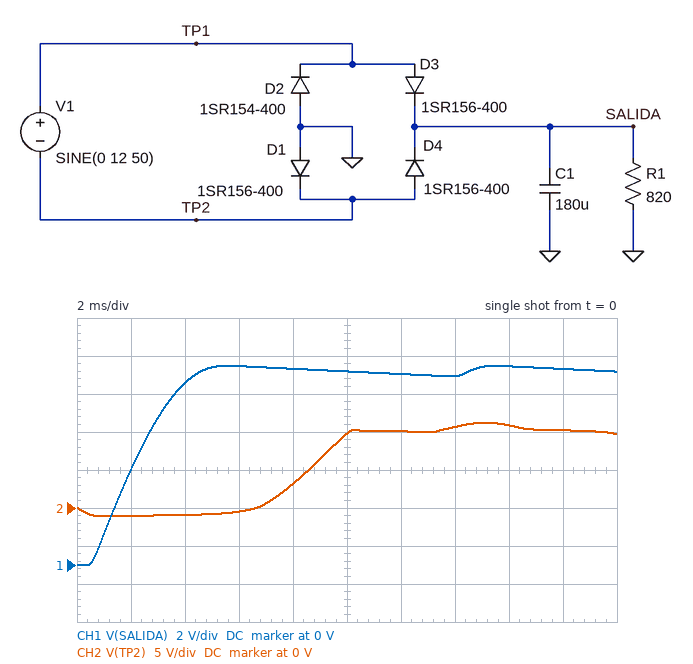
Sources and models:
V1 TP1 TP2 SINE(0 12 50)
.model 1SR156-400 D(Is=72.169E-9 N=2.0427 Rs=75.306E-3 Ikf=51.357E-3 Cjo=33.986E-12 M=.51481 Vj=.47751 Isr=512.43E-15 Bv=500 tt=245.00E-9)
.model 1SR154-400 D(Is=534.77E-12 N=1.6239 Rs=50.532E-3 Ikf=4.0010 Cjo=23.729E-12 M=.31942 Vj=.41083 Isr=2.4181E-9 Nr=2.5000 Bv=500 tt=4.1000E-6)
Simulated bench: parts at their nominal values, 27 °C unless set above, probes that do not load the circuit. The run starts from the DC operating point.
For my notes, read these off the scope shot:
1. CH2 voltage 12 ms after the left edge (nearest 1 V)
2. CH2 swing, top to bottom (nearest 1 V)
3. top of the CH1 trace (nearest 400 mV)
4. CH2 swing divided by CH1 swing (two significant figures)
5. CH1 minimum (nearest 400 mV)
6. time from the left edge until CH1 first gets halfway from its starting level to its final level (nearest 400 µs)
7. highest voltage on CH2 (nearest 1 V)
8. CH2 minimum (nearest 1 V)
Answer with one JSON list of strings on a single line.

["10 V", "12 V", "10.4 V", "1.2", "0 V", "2.0 ms", "11 V", "-1 V"]
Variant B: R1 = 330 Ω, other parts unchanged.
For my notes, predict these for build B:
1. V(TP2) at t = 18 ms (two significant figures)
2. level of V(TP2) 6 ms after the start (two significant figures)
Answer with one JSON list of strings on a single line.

["9.9 V", "-520 mV"]
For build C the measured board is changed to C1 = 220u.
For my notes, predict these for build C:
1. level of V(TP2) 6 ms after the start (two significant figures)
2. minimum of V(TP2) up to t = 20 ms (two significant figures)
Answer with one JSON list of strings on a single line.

["-480 mV", "-1.1 V"]
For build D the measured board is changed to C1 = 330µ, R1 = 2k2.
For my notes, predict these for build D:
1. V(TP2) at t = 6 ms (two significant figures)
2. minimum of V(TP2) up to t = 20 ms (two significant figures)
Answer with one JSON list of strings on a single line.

["-500 mV", "-1.1 V"]
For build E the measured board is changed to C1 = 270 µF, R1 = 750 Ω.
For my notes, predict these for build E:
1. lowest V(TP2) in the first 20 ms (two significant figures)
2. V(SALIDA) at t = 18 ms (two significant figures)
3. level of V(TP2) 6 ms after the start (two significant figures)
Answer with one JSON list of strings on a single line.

["-1.1 V", "10 V", "-500 mV"]
